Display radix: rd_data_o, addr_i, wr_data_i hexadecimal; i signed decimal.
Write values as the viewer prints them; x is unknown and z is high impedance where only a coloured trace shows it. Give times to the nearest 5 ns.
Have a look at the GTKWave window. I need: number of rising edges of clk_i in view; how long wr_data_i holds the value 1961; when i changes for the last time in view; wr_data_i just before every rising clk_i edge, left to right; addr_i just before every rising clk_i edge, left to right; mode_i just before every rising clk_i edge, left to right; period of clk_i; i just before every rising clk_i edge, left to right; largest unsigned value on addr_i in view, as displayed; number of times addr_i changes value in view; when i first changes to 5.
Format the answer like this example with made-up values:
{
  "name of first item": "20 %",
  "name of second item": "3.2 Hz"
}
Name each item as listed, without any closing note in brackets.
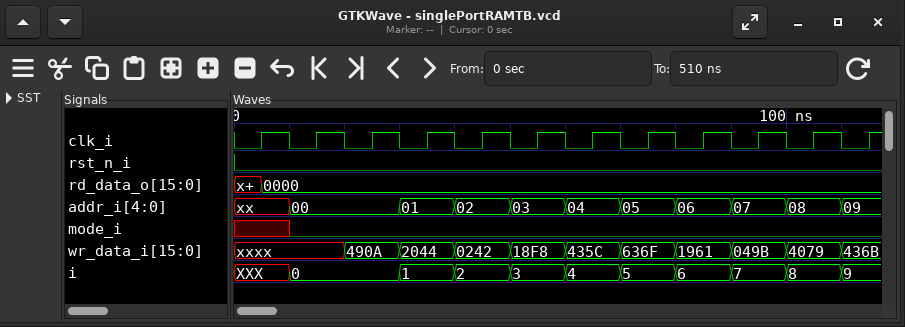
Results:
{
  "number of rising edges of clk_i in view": "12",
  "how long wr_data_i holds the value 1961": "10 ns",
  "when i changes for the last time in view": "110 ns",
  "wr_data_i just before every rising clk_i edge, left to right": "xxxx, xxxx, 490A, 2044, 0242, 18F8, 435C, 636F, 1961, 049B, 4079, 436B",
  "addr_i just before every rising clk_i edge, left to right": "xx, 00, 00, 01, 02, 03, 04, 05, 06, 07, 08, 09",
  "mode_i just before every rising clk_i edge, left to right": "x 0 0 0 0 0 0 0 0 0 0 0",
  "period of clk_i": "10 ns",
  "i just before every rising clk_i edge, left to right": "XXX, 0, 0, 1, 2, 3, 4, 5, 6, 7, 8, 9",
  "largest unsigned value on addr_i in view, as displayed": "09",
  "number of times addr_i changes value in view": "10",
  "when i first changes to 5": "70 ns"
}
